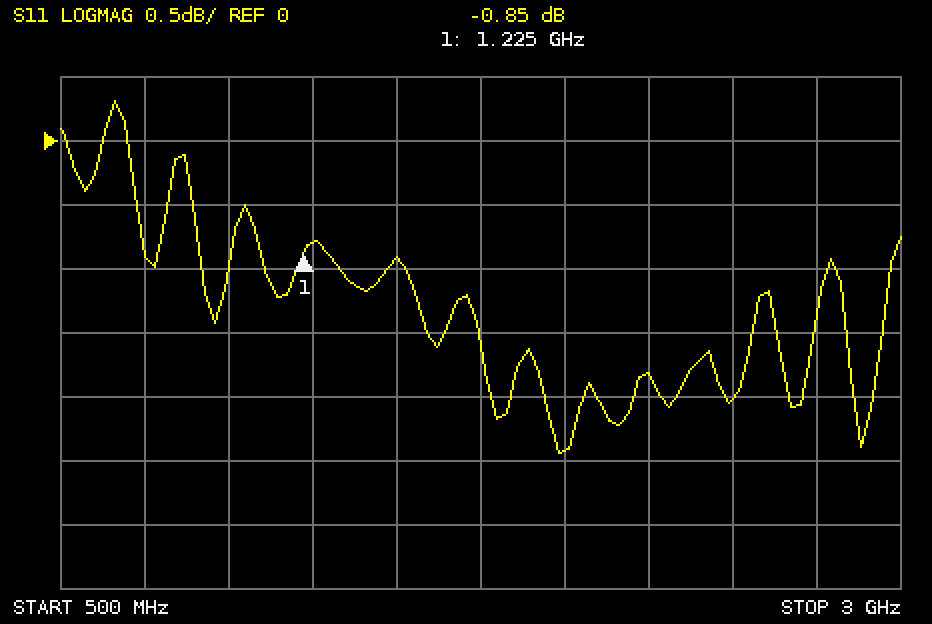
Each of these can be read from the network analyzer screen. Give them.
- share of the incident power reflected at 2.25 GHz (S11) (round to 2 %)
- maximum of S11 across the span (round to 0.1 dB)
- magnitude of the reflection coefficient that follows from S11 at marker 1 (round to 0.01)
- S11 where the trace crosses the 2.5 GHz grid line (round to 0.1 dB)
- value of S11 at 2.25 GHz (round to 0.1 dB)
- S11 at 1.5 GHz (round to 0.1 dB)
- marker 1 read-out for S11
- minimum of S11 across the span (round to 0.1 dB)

66 %
0.3 dB
0.91
-2.0 dB
-1.8 dB
-0.9 dB
-0.85 dB
-2.4 dB
